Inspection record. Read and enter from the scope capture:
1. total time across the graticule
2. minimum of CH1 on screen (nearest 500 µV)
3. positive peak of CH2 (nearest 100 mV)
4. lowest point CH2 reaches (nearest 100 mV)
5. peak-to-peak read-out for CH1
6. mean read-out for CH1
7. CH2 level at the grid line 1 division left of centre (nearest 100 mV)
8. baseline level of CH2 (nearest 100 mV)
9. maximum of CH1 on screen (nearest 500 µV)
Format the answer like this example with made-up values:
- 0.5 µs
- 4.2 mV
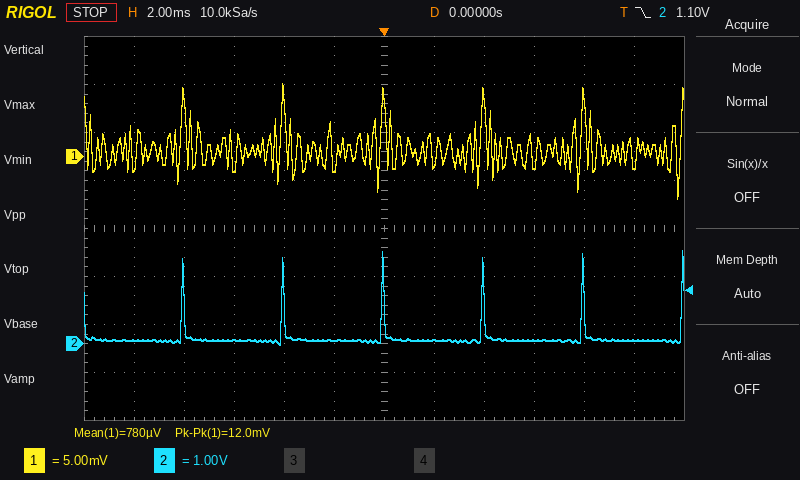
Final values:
- 24 ms
- -4.5 mV
- 1.9 V
- 0.0 V
- 12.0 mV
- 780 µV
- 100 mV
- 100 mV
- 7.5 mV
